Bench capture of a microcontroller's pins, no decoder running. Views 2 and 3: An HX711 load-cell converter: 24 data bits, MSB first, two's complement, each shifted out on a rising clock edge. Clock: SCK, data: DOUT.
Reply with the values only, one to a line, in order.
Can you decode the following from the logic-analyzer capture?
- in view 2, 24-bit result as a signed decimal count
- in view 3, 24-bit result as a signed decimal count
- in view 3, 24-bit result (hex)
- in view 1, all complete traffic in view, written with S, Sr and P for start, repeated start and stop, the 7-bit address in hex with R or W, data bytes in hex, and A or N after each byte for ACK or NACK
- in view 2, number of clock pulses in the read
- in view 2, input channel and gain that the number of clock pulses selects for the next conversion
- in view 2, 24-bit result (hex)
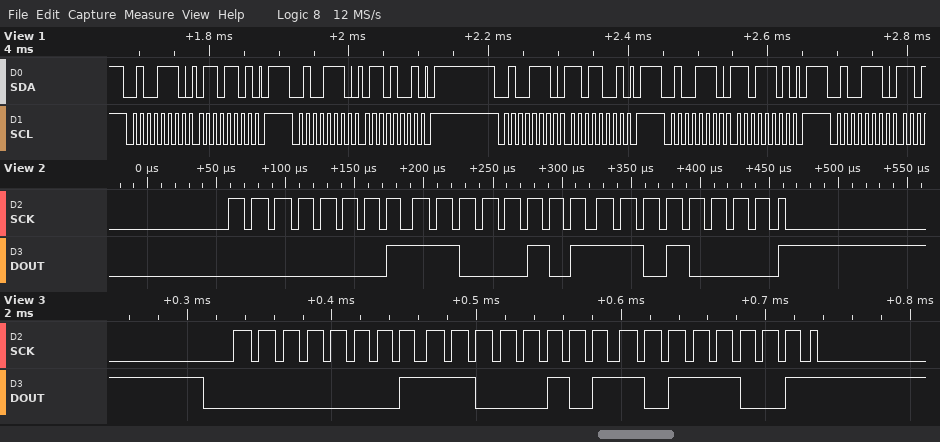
116176
116153
0x01C5B9
S 27W A 6D A P S 27W A 69 A P S 27W A D9 A P S 27W A DD A P S 27W A
25
channel A, gain 128
0x01C5D0
